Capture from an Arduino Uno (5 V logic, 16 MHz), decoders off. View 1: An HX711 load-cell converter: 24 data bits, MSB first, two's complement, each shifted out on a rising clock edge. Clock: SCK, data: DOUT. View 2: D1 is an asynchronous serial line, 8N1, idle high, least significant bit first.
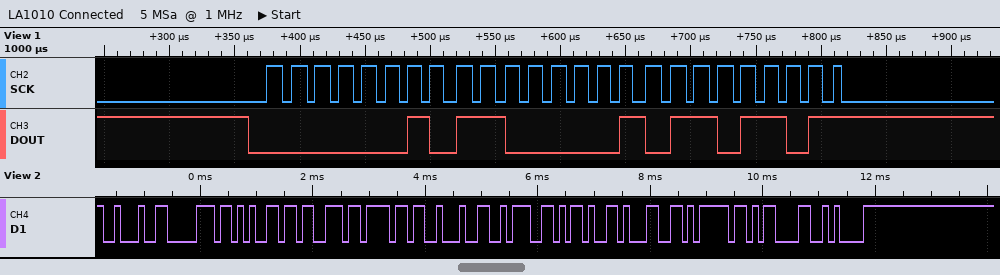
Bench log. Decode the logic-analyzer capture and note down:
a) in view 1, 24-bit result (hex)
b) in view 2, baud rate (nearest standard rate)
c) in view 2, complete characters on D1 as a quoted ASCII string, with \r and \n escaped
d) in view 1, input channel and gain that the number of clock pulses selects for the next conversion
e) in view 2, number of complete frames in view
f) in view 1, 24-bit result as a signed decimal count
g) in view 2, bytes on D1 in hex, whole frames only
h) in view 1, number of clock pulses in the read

0x02C16D
9600 baud
"\"peso\":-1}\r\n"
channel A, gain 128
12
180589
22 70 65 73 6F 22 3A 2D 31 7D 0D 0A
25
